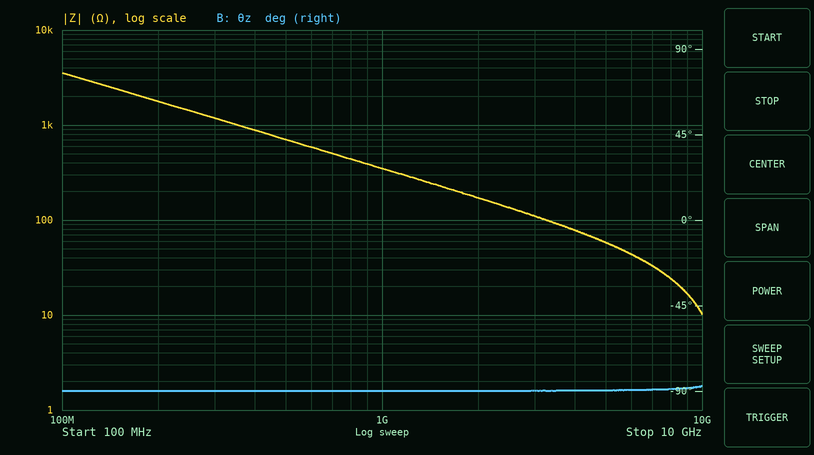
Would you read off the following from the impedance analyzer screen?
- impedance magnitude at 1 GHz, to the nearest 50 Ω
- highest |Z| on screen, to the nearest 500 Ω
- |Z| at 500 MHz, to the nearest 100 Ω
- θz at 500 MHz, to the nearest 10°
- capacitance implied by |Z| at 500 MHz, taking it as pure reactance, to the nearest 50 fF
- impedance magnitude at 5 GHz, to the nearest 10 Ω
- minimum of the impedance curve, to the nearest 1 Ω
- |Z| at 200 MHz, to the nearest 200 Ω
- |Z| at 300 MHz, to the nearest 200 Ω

350 Ω
3.5 kΩ
700 Ω
-90°
450 fF
60 Ω
10 Ω
1.8 kΩ
1.2 kΩ
